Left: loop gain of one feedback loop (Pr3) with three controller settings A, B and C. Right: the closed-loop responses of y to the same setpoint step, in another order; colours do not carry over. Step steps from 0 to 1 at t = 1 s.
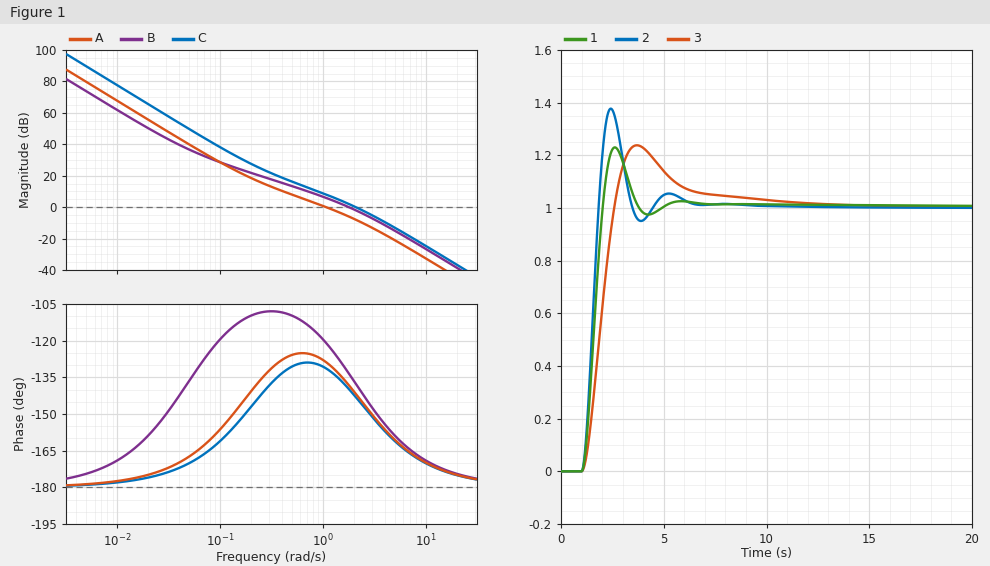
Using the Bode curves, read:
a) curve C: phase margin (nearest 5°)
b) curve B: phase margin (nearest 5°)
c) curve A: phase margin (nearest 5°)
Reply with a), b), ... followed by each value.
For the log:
a) 35°
b) 45°
c) 50°
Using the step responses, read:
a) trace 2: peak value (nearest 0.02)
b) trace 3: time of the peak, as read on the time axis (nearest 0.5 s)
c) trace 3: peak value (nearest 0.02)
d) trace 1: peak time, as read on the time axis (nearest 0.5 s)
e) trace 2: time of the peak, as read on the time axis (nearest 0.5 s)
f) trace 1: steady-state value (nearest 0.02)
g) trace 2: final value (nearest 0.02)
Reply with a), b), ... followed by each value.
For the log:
a) 1.38
b) 3.5 s
c) 1.24
d) 2.5 s
e) 2.5 s
f) 1.00
g) 1.00
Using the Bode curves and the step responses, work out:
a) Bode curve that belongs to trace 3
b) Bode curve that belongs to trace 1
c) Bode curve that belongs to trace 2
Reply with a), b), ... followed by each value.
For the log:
a) A
b) B
c) C
